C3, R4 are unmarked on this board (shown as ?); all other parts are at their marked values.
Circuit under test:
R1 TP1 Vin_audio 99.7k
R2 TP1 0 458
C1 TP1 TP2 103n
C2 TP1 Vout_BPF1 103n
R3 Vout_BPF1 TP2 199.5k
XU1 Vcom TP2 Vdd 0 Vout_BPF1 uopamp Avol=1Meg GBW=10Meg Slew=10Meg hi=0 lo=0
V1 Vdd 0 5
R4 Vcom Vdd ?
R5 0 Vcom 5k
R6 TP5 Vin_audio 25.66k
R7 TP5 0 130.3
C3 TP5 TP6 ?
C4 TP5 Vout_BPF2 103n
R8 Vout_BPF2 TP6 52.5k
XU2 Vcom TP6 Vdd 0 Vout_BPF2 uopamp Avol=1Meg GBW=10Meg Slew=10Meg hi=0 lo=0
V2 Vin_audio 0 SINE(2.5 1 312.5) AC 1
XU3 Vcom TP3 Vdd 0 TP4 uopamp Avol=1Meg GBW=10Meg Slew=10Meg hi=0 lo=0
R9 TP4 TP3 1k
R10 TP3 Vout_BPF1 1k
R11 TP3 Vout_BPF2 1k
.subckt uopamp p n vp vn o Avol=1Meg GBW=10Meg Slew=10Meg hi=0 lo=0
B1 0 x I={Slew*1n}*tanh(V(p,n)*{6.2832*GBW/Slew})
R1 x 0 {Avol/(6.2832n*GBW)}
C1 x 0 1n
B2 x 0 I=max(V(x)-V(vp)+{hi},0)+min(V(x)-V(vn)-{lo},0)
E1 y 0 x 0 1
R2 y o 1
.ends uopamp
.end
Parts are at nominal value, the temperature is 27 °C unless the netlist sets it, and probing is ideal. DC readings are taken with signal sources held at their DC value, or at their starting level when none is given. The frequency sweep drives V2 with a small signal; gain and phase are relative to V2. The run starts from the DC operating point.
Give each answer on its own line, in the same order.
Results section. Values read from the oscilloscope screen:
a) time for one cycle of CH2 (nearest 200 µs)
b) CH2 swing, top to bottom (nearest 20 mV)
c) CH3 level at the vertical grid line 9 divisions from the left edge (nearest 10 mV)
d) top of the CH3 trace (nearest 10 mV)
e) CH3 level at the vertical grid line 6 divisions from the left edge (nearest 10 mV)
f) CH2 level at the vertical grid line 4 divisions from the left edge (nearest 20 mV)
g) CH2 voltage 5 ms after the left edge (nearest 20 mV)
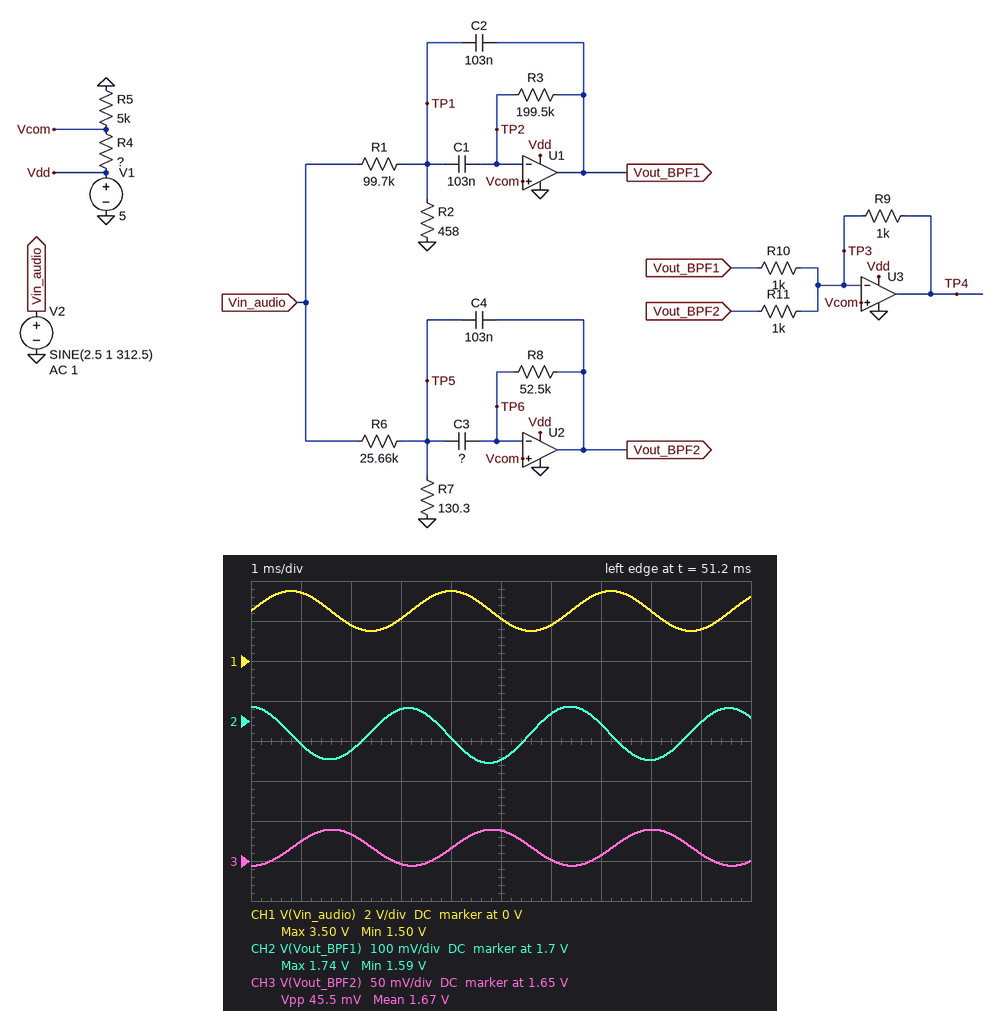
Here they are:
3.2 ms
140 mV
1.66 V
1.69 V
1.65 V
1.66 V
1.60 V
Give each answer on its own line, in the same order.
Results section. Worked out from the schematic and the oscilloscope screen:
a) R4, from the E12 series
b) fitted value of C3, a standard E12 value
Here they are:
10 kΩ
39 nF
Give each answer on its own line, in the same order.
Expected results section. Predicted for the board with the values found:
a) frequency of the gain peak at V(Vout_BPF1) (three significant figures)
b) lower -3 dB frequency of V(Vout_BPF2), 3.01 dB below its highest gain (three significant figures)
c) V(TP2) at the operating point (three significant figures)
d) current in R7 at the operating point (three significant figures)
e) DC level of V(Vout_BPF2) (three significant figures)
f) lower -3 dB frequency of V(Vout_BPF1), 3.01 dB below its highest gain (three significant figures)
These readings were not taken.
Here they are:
162 Hz
910 Hz
1.67 V
96.9 µA
1.67 V
154 Hz
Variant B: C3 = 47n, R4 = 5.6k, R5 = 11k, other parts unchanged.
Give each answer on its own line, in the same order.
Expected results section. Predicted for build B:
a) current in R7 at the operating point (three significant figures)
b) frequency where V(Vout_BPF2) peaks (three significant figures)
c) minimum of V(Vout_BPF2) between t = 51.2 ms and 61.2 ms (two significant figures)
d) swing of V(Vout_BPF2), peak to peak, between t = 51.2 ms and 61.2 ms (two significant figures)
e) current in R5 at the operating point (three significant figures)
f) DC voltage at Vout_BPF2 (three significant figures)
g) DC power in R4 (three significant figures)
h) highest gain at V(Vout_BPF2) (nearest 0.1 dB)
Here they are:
96.9 µA
876 Hz
3.3 V
56 mV
301 µA
3.31 V
508 µW
-3.9 dB
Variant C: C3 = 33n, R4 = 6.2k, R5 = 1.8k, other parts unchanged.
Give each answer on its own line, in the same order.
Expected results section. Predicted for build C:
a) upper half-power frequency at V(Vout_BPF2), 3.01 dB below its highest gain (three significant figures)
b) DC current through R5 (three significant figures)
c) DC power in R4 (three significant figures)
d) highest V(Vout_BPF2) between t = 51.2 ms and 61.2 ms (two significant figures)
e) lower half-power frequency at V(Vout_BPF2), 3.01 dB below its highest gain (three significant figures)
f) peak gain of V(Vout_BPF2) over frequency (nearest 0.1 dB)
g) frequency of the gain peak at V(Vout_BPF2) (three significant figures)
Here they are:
1.11 kHz
625 µA
2.42 mW
1.1 V
987 Hz
-6.1 dB
1.05 kHz
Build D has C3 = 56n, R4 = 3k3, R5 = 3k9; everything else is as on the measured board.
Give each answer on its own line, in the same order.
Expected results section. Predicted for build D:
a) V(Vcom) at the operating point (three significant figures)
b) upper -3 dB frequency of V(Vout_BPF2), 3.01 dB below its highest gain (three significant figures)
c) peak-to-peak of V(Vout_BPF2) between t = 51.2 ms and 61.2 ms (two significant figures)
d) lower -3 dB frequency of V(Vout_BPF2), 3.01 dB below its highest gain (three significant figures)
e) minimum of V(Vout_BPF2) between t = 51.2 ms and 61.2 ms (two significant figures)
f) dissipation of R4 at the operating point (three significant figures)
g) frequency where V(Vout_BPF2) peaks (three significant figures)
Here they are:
2.71 V
846 Hz
69 mV
762 Hz
2.7 V
1.59 mW
803 Hz
